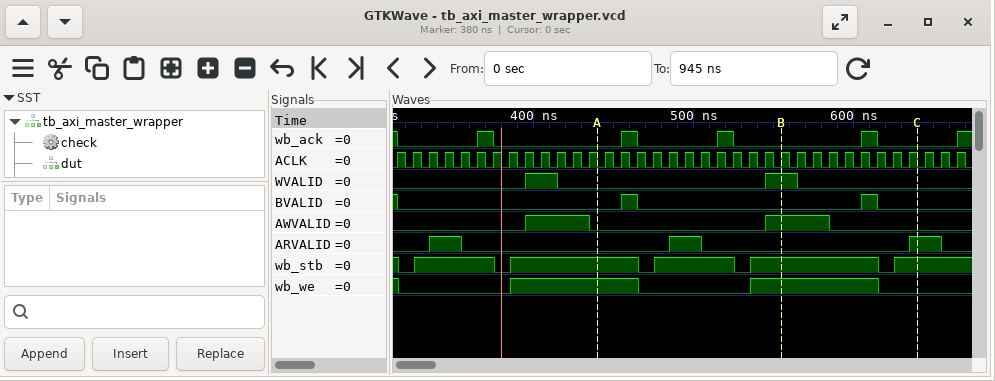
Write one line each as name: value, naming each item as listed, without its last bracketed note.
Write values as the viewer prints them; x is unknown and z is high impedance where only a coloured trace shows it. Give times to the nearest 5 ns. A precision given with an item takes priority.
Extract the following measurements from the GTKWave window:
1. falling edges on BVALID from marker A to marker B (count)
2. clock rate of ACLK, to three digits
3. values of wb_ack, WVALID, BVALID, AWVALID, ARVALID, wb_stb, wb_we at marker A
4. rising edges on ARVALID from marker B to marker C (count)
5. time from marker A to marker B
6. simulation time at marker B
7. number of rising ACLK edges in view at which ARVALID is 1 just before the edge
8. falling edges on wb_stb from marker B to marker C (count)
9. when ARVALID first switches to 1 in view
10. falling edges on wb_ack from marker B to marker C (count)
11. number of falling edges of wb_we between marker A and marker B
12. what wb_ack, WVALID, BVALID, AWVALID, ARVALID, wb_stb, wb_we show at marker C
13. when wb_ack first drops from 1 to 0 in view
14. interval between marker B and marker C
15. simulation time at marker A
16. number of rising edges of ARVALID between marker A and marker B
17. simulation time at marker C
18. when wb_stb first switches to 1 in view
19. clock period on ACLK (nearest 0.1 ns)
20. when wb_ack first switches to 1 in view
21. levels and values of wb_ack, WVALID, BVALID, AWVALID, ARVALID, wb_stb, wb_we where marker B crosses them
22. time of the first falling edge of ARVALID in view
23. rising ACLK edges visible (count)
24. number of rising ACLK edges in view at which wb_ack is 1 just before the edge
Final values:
falling edges on BVALID from marker A to marker B: 1
clock rate of ACLK, to three digits: 100 MHz
values of wb_ack, WVALID, BVALID, AWVALID, ARVALID, wb_stb, wb_we at marker A: wb_ack=0, WVALID=0, BVALID=0, AWVALID=0, ARVALID=0, wb_stb=1, wb_we=1
rising edges on ARVALID from marker B to marker C: 1
time from marker A to marker B: 115 ns
simulation time at marker B: 555 ns
number of rising ACLK edges in view at which ARVALID is 1 just before the edge: 6
falling edges on wb_stb from marker B to marker C: 1
when ARVALID first switches to 1 in view: 335 ns
falling edges on wb_ack from marker B to marker C: 1
number of falling edges of wb_we between marker A and marker B: 1
what wb_ack, WVALID, BVALID, AWVALID, ARVALID, wb_stb, wb_we show at marker C: wb_ack=0, WVALID=0, BVALID=0, AWVALID=0, ARVALID=1, wb_stb=1, wb_we=0
when wb_ack first drops from 1 to 0 in view: 315 ns
interval between marker B and marker C: 85 ns
simulation time at marker A: 440 ns
number of rising edges of ARVALID between marker A and marker B: 1
simulation time at marker C: 640 ns
when wb_stb first switches to 1 in view: 325 ns
clock period on ACLK: 10 ns
when wb_ack first switches to 1 in view: 365 ns
levels and values of wb_ack, WVALID, BVALID, AWVALID, ARVALID, wb_stb, wb_we where marker B crosses them: wb_ack=0, WVALID=1, BVALID=0, AWVALID=1, ARVALID=0, wb_stb=1, wb_we=1
time of the first falling edge of ARVALID in view: 355 ns
rising ACLK edges visible: 36
number of rising ACLK edges in view at which wb_ack is 1 just before the edge: 5
